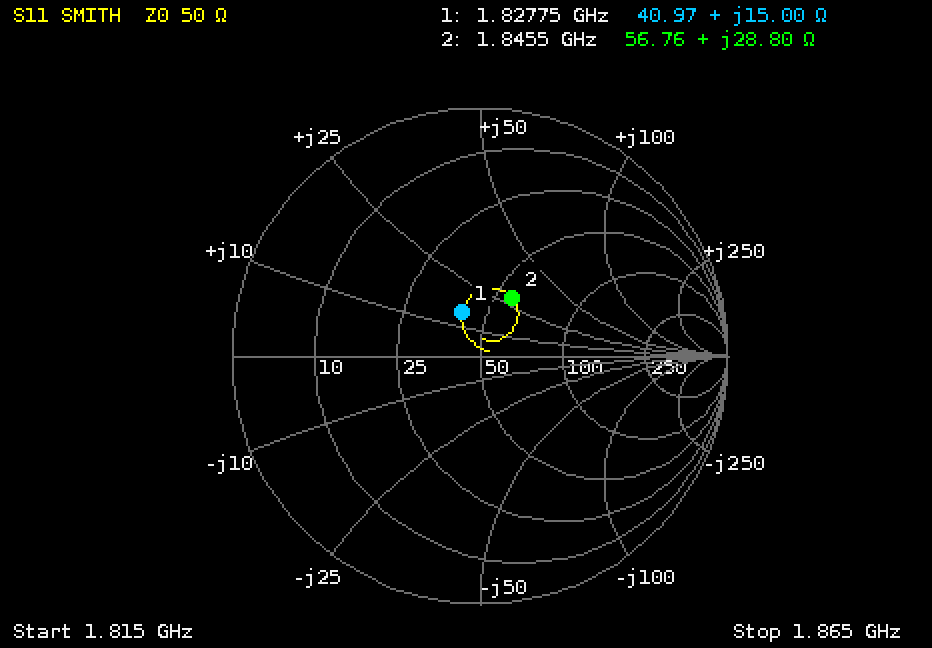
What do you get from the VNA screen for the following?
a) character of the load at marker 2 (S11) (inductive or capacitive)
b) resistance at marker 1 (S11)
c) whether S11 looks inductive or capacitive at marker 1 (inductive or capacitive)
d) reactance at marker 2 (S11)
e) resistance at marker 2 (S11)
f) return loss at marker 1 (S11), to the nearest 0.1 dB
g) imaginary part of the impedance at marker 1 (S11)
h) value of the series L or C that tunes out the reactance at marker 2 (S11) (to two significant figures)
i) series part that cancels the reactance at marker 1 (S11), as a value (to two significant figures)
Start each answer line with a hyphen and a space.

- inductive
- 40.97 Ω
- inductive
- +28.80 Ω
- 56.76 Ω
- 14.4 dB
- +15.00 Ω
- 3.0 pF
- 5.8 pF
